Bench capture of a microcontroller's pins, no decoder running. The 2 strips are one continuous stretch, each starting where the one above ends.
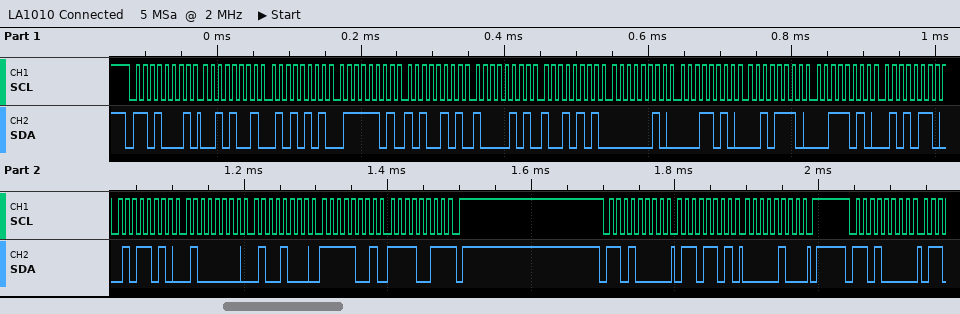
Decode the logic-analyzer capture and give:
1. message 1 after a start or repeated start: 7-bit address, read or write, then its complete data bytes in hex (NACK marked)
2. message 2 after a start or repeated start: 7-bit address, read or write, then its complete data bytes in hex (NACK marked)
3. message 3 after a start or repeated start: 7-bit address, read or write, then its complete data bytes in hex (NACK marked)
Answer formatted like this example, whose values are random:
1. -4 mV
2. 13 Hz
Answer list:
1. 0x68 read: 29 55 7D A5 85 95 02 1A 2E 3A 56 5A 40 48 F9 F3 NACK
2. 0x68 write: 6D 04
3. 0x68 write
